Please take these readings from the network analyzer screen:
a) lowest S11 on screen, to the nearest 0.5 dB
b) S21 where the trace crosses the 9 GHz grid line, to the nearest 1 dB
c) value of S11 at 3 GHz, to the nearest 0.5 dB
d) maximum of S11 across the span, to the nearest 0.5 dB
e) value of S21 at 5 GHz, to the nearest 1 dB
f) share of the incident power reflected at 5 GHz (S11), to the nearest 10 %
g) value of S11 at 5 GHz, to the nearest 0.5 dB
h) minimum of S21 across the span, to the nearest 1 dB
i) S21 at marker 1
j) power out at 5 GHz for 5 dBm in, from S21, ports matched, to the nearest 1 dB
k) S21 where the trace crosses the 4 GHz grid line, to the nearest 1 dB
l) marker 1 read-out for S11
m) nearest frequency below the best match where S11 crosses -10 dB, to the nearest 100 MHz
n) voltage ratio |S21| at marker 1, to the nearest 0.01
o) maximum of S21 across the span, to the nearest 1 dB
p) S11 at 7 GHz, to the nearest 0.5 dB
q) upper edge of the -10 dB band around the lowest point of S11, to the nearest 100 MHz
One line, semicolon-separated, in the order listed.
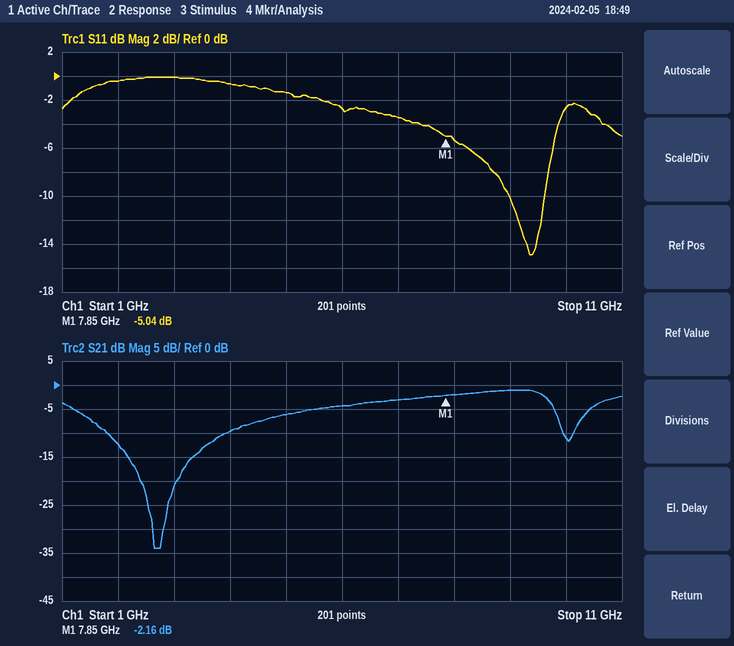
-15.0 dB; -1 dB; 0.0 dB; 0.0 dB; -6 dB; 70 %; -1.5 dB; -34 dB; -2.16 dB; -1 dBm; -10 dB; -5.04 dB; 9.0 GHz; 0.78; -1 dB; -3.5 dB; 9.6 GHz
